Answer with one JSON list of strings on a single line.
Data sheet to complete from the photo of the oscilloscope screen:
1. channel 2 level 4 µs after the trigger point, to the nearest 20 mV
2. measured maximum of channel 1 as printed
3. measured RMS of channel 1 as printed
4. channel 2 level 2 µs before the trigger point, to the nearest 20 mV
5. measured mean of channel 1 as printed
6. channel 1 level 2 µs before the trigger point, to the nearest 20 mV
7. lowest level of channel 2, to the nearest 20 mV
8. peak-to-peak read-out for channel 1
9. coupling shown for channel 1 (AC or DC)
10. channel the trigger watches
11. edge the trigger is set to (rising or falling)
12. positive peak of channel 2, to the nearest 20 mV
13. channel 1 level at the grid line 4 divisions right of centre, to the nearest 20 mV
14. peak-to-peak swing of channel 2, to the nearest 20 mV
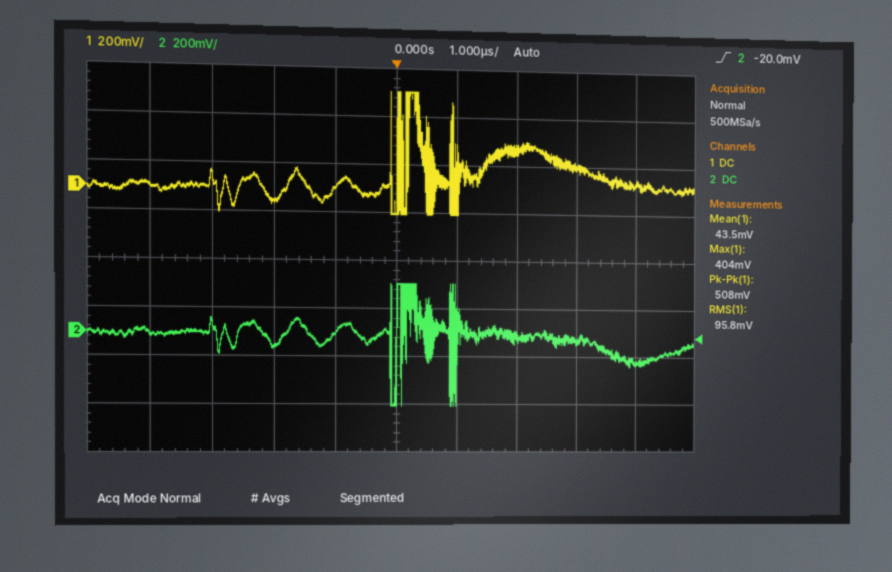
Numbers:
["-120 mV", "404 mV", "95.8 mV", "-60 mV", "43.5 mV", "-60 mV", "-300 mV", "508 mV", "DC", "channel 2", "rising", "200 mV", "40 mV", "500 mV"]
